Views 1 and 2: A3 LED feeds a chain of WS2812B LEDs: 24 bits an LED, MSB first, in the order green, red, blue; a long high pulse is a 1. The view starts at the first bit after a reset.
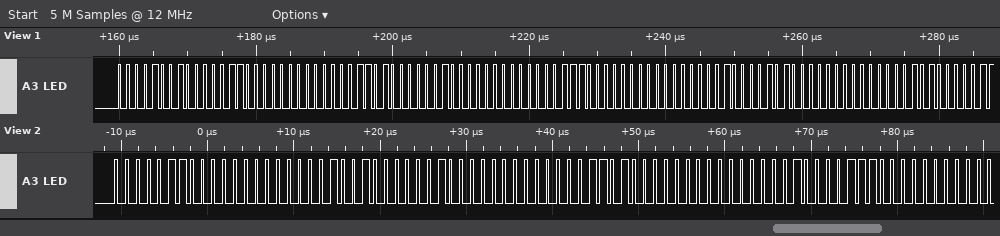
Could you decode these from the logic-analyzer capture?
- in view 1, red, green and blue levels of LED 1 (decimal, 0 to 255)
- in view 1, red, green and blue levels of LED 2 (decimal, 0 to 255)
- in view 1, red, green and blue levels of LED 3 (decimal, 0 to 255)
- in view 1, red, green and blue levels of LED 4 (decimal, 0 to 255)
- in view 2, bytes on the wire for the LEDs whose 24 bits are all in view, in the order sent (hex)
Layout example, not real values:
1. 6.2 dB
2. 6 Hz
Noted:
1. 6, 9, 0
2. 2, 13, 0
3. 0, 14, 1
4. 0, 10, 5
5. 06 00 09 02 00 0D 00 01 0E
